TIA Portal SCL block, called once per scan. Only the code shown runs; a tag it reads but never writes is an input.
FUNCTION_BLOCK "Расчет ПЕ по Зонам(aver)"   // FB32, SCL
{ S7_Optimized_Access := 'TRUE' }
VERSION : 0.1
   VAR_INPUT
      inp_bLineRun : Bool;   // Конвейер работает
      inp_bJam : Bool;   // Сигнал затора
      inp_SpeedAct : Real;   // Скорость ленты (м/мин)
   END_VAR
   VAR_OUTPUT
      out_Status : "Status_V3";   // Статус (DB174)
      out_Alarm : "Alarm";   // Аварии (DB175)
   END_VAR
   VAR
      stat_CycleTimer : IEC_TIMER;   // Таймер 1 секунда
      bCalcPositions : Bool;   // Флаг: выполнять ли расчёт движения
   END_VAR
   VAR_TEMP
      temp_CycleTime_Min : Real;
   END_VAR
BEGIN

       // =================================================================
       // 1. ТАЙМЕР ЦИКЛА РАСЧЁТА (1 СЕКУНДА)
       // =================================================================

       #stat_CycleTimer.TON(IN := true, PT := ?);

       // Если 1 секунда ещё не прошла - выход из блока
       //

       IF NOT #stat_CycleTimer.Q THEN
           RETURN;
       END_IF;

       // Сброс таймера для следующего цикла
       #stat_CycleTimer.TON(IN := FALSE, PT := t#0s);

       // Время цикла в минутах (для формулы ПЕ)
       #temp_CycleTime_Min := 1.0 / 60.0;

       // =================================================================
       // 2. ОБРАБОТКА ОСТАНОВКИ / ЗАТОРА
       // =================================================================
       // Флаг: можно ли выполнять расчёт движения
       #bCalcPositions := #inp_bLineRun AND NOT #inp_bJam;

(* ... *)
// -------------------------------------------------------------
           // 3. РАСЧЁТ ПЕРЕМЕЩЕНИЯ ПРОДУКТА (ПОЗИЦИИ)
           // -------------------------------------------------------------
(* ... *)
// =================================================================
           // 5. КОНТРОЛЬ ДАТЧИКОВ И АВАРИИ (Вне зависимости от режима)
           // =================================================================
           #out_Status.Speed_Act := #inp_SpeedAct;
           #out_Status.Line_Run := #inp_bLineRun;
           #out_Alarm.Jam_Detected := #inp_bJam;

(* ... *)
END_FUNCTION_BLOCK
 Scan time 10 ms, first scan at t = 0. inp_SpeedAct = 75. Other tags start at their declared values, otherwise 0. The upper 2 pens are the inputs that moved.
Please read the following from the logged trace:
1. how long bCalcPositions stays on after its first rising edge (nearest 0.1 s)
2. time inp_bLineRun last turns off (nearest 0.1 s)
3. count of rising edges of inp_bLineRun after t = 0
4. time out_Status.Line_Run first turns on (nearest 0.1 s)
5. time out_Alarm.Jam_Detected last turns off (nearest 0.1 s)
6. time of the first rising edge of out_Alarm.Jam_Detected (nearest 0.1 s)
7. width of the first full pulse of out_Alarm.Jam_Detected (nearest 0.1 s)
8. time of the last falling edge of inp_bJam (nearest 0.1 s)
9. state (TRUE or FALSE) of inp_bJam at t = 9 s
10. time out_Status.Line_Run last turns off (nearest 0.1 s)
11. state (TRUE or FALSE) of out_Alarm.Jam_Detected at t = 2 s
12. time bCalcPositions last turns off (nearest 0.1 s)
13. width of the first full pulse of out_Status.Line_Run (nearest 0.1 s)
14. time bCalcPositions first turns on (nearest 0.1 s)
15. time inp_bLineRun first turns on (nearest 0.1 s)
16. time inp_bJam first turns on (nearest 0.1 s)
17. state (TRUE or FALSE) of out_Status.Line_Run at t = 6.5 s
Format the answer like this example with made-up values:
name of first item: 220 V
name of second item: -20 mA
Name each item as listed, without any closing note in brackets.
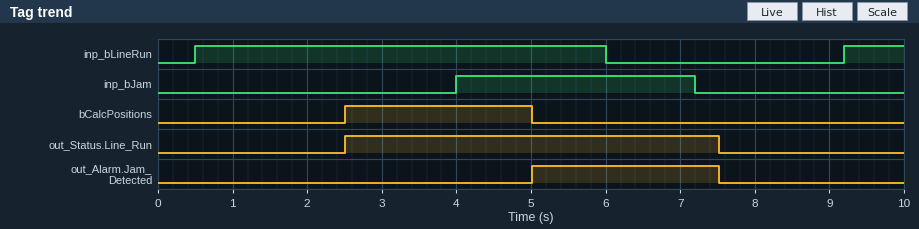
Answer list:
how long bCalcPositions stays on after its first rising edge: 2.5 s
time inp_bLineRun last turns off: 6.0 s
count of rising edges of inp_bLineRun after t = 0: 2
time out_Status.Line_Run first turns on: 2.5 s
time out_Alarm.Jam_Detected last turns off: 7.5 s
time of the first rising edge of out_Alarm.Jam_Detected: 5.0 s
width of the first full pulse of out_Alarm.Jam_Detected: 2.5 s
time of the last falling edge of inp_bJam: 7.2 s
state (TRUE or FALSE) of inp_bJam at t = 9 s: FALSE
time out_Status.Line_Run last turns off: 7.5 s
state (TRUE or FALSE) of out_Alarm.Jam_Detected at t = 2 s: FALSE
time bCalcPositions last turns off: 5.0 s
width of the first full pulse of out_Status.Line_Run: 5.0 s
time bCalcPositions first turns on: 2.5 s
time inp_bLineRun first turns on: 0.5 s
time inp_bJam first turns on: 4.0 s
state (TRUE or FALSE) of out_Status.Line_Run at t = 6.5 s: TRUE
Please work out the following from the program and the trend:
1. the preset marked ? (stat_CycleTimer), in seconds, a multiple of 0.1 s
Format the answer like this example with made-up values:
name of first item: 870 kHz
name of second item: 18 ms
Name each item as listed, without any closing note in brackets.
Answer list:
the preset marked ? (stat_CycleTimer), in seconds, a multiple of 0.1 s: 2.5 s
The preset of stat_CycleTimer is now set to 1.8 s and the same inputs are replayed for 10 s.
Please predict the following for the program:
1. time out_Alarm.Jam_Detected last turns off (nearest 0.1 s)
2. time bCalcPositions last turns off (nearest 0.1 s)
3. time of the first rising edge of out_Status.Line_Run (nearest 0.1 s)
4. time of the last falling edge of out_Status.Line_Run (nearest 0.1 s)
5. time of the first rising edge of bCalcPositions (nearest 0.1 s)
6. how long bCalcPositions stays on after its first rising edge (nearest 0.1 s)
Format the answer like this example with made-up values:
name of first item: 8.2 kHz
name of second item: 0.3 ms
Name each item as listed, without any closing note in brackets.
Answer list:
time out_Alarm.Jam_Detected last turns off: 7.2 s
time bCalcPositions last turns off: 5.4 s
time of the first rising edge of out_Status.Line_Run: 1.8 s
time of the last falling edge of out_Status.Line_Run: 7.2 s
time of the first rising edge of bCalcPositions: 1.8 s
how long bCalcPositions stays on after its first rising edge: 3.6 s
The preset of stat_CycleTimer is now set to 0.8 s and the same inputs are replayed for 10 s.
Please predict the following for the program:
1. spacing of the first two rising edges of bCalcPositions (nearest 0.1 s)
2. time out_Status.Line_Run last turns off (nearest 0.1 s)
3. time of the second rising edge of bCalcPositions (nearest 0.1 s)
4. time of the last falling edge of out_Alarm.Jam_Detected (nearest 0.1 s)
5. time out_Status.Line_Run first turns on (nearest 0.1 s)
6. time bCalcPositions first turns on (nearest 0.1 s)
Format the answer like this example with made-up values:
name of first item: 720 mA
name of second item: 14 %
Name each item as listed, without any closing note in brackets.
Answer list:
spacing of the first two rising edges of bCalcPositions: 8.9 s
time out_Status.Line_Run last turns off: 6.5 s
time of the second rising edge of bCalcPositions: 9.7 s
time of the last falling edge of out_Alarm.Jam_Detected: 7.3 s
time out_Status.Line_Run first turns on: 0.8 s
time bCalcPositions first turns on: 0.8 s
